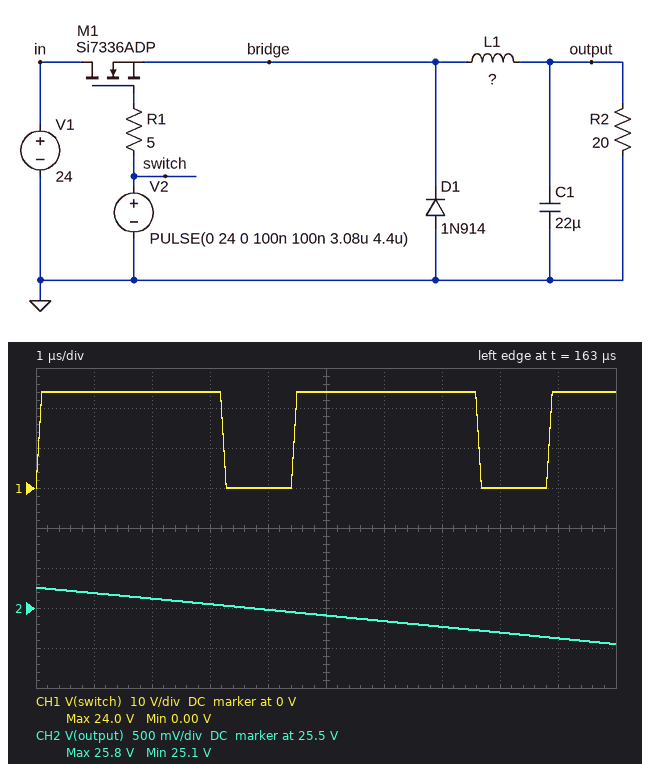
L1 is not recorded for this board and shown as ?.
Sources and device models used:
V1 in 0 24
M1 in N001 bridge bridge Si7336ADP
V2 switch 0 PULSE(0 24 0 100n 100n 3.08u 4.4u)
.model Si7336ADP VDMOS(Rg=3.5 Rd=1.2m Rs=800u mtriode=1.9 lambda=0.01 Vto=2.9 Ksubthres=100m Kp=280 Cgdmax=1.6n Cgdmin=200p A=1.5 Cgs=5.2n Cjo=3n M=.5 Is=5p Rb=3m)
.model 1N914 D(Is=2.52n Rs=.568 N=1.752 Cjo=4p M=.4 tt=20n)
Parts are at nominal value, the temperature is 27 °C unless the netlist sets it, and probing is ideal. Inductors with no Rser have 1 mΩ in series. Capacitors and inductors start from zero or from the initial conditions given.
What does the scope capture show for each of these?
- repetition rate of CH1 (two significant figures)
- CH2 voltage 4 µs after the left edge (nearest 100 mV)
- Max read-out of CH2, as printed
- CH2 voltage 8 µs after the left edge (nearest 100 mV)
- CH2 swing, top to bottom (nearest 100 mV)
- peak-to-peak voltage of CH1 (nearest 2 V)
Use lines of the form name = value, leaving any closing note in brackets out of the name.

repetition rate of CH1 = 230 kHz
CH2 voltage 4 µs after the left edge = 25.5 V
Max read-out of CH2, as printed = 25.8 V
CH2 voltage 8 µs after the left edge = 25.2 V
CH2 swing, top to bottom = 700 mV
peak-to-peak voltage of CH1 = 24 V
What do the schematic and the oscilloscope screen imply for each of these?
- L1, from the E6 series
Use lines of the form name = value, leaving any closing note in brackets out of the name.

L1, from the E6 series = 100 µH
